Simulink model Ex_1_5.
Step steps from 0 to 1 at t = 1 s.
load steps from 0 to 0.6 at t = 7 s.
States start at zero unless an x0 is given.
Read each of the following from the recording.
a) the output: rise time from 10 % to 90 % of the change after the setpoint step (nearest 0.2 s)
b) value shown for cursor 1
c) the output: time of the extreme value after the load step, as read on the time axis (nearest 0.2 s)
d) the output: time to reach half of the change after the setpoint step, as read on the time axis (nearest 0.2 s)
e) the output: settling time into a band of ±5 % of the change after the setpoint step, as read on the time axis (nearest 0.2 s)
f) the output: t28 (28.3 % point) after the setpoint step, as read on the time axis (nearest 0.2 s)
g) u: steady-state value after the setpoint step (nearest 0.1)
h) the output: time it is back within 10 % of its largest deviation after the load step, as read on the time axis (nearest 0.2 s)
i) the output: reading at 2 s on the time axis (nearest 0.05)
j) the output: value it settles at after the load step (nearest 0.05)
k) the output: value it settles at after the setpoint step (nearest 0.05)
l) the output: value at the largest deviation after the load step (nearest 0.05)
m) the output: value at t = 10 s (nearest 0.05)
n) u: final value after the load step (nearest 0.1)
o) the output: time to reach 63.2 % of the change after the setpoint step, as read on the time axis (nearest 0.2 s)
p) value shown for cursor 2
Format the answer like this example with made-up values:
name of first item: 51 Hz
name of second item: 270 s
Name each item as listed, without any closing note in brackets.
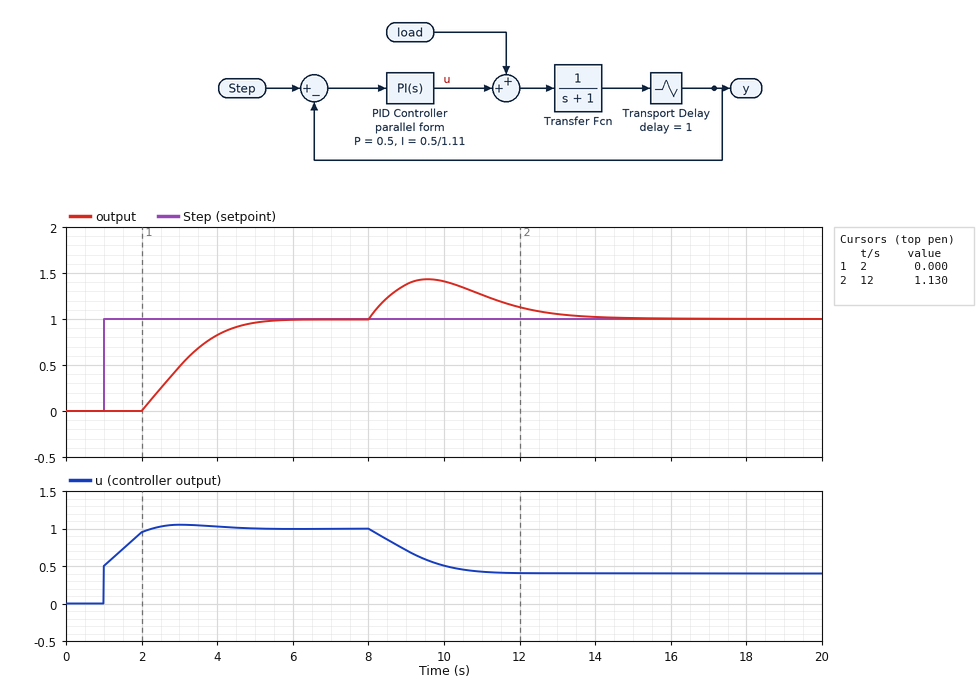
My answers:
the output: rise time from 10 % to 90 % of the change after the setpoint step: 2.2 s
value shown for cursor 1: 0.000
the output: time of the extreme value after the load step, as read on the time axis: 9.6 s
the output: time to reach half of the change after the setpoint step, as read on the time axis: 3.0 s
the output: settling time into a band of ±5 % of the change after the setpoint step, as read on the time axis: 4.8 s
the output: t28 (28.3 % point) after the setpoint step, as read on the time axis: 2.6 s
u: steady-state value after the setpoint step: 1.0
the output: time it is back within 10 % of its largest deviation after the load step, as read on the time axis: 13.2 s
the output: reading at 2 s on the time axis: 0.00
the output: value it settles at after the load step: 1.00
the output: value it settles at after the setpoint step: 1.00
the output: value at the largest deviation after the load step: 1.45
the output: value at t = 10 s: 1.40
u: final value after the load step: 0.4
the output: time to reach 63.2 % of the change after the setpoint step, as read on the time axis: 3.4 s
value shown for cursor 2: 1.130
